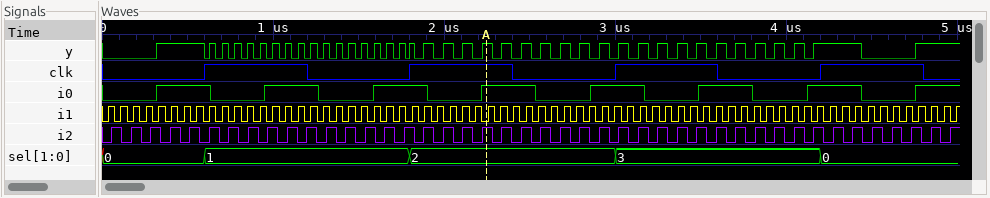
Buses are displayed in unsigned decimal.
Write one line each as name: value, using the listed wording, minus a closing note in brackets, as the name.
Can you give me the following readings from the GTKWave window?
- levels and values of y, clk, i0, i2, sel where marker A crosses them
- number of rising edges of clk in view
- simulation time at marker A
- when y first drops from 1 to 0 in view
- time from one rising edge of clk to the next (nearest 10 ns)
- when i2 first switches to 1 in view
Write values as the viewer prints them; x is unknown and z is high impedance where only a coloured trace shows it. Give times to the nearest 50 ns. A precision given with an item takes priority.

levels and values of y, clk, i0, i2, sel where marker A crosses them: y=1, clk=1, i0=1, i2=1, sel=2
number of rising edges of clk in view: 4
simulation time at marker A: 2250 ns
when y first drops from 1 to 0 in view: 600 ns
time from one rising edge of clk to the next: 1200 ns
when i2 first switches to 1 in view: 50 ns
